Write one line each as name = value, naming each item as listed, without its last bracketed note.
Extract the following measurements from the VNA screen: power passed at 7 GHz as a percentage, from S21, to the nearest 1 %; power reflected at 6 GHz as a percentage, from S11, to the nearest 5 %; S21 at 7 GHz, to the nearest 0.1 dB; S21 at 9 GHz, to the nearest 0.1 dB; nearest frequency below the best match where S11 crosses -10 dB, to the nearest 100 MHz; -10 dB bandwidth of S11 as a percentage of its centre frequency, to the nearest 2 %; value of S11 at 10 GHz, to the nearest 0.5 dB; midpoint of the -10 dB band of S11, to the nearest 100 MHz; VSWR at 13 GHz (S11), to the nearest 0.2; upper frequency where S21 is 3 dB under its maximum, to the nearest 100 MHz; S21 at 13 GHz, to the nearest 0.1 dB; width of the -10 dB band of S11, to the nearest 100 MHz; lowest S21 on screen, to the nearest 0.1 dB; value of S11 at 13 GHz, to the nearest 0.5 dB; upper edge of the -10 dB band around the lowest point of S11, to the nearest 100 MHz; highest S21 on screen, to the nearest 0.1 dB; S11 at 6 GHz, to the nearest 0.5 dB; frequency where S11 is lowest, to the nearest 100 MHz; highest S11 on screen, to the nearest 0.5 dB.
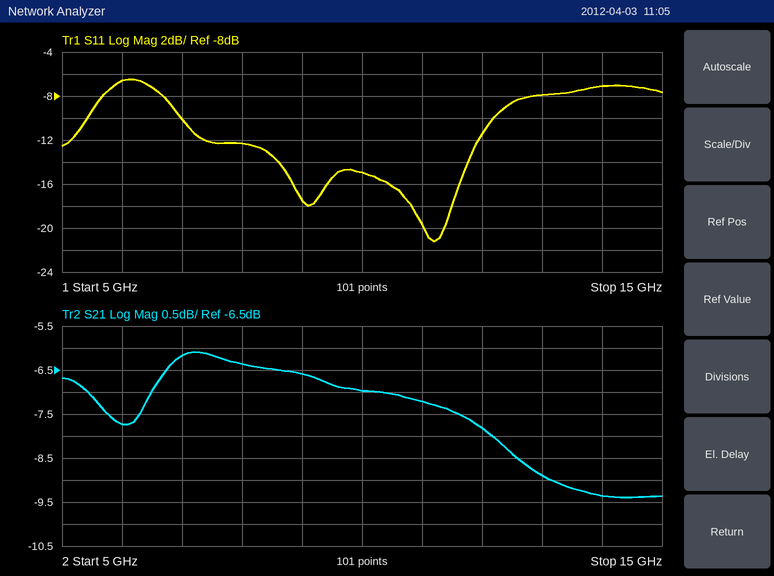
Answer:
power passed at 7 GHz as a percentage, from S21, to the nearest 1 % = 24 %
power reflected at 6 GHz as a percentage, from S11, to the nearest 5 % = 20 %
S21 at 7 GHz, to the nearest 0.1 dB = -6.2 dB
S21 at 9 GHz, to the nearest 0.1 dB = -6.6 dB
nearest frequency below the best match where S11 crosses -10 dB, to the nearest 100 MHz = 7.0 GHz
-10 dB bandwidth of S11 as a percentage of its centre frequency, to the nearest 2 % = 54 %
value of S11 at 10 GHz, to the nearest 0.5 dB = -15.0 dB
midpoint of the -10 dB band of S11, to the nearest 100 MHz = 9.6 GHz
VSWR at 13 GHz (S11), to the nearest 0.2 = 2.4
upper frequency where S21 is 3 dB under its maximum, to the nearest 100 MHz = 13.3 GHz
S21 at 13 GHz, to the nearest 0.1 dB = -8.9 dB
width of the -10 dB band of S11, to the nearest 100 MHz = 5.2 GHz
lowest S21 on screen, to the nearest 0.1 dB = -9.4 dB
value of S11 at 13 GHz, to the nearest 0.5 dB = -8.0 dB
upper edge of the -10 dB band around the lowest point of S11, to the nearest 100 MHz = 12.2 GHz
highest S21 on screen, to the nearest 0.1 dB = -6.1 dB
S11 at 6 GHz, to the nearest 0.5 dB = -6.5 dB
frequency where S11 is lowest, to the nearest 100 MHz = 11.2 GHz
highest S11 on screen, to the nearest 0.5 dB = -6.5 dB
